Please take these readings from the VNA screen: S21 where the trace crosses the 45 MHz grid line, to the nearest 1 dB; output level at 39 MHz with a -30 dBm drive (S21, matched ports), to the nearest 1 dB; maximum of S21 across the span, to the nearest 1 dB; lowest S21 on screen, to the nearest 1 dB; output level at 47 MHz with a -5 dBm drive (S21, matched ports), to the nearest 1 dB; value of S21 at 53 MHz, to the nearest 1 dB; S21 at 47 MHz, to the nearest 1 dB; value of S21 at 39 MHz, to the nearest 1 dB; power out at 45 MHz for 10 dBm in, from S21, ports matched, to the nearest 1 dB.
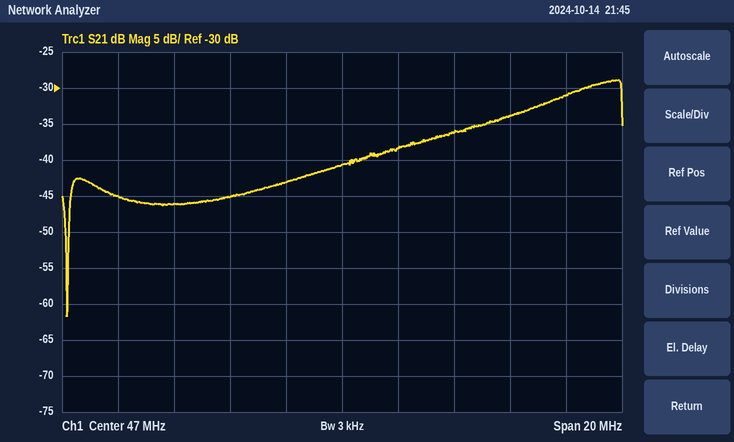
-43 dB
-75 dBm
-29 dB
-62 dB
-46 dBm
-34 dB
-41 dB
-45 dB
-33 dBm
